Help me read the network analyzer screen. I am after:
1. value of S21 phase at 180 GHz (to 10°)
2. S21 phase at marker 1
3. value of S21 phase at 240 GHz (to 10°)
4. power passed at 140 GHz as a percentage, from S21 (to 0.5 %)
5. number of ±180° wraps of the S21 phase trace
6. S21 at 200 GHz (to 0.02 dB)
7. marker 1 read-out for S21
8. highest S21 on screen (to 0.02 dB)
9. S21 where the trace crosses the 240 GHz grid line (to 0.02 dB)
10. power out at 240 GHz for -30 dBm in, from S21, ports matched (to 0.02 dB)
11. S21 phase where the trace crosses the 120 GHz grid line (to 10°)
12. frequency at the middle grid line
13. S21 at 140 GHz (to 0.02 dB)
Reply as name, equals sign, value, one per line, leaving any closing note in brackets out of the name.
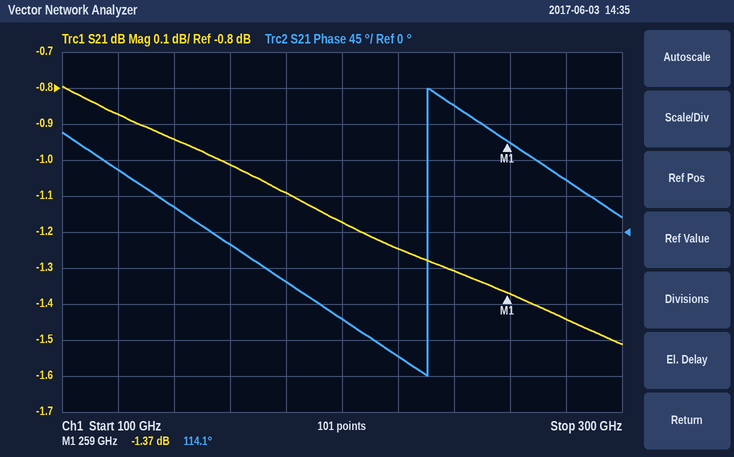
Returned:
value of S21 phase at 180 GHz = -60°
S21 phase at marker 1 = 114.1°
value of S21 phase at 240 GHz = 160°
power passed at 140 GHz as a percentage, from S21 = 80.5 %
number of ±180° wraps of the S21 phase trace = 1
S21 at 200 GHz = -1.18 dB
marker 1 read-out for S21 = -1.37 dB
highest S21 on screen = -0.80 dB
S21 where the trace crosses the 240 GHz grid line = -1.30 dB
power out at 240 GHz for -30 dBm in, from S21, ports matched = -31.30 dBm
S21 phase where the trace crosses the 120 GHz grid line = 80°
frequency at the middle grid line = 200 GHz
S21 at 140 GHz = -0.94 dB
